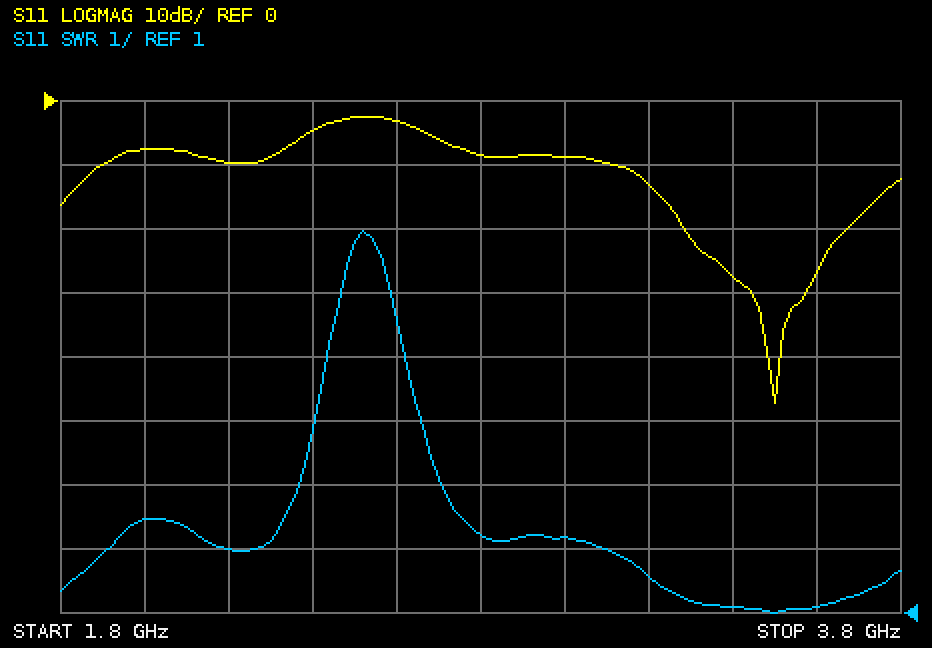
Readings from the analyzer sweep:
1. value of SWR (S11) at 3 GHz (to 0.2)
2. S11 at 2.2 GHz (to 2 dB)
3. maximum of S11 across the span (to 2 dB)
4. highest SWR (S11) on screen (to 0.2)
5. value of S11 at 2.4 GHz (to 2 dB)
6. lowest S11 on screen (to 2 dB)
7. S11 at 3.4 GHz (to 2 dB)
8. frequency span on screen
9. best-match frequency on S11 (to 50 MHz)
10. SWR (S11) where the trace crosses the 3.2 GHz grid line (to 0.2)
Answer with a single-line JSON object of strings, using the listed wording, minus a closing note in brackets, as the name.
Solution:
{"value of SWR (S11) at 3 GHz": "2.2", "S11 at 2.2 GHz": "-10 dB", "maximum of S11 across the span": "-2 dB", "highest SWR (S11) on screen": "7.0", "value of S11 at 2.4 GHz": "-4 dB", "lowest S11 on screen": "-48 dB", "S11 at 3.4 GHz": "-28 dB", "frequency span on screen": "2 GHz", "best-match frequency on S11": "3.50 GHz", "SWR (S11) where the trace crosses the 3.2 GHz grid line": "1.6"}
